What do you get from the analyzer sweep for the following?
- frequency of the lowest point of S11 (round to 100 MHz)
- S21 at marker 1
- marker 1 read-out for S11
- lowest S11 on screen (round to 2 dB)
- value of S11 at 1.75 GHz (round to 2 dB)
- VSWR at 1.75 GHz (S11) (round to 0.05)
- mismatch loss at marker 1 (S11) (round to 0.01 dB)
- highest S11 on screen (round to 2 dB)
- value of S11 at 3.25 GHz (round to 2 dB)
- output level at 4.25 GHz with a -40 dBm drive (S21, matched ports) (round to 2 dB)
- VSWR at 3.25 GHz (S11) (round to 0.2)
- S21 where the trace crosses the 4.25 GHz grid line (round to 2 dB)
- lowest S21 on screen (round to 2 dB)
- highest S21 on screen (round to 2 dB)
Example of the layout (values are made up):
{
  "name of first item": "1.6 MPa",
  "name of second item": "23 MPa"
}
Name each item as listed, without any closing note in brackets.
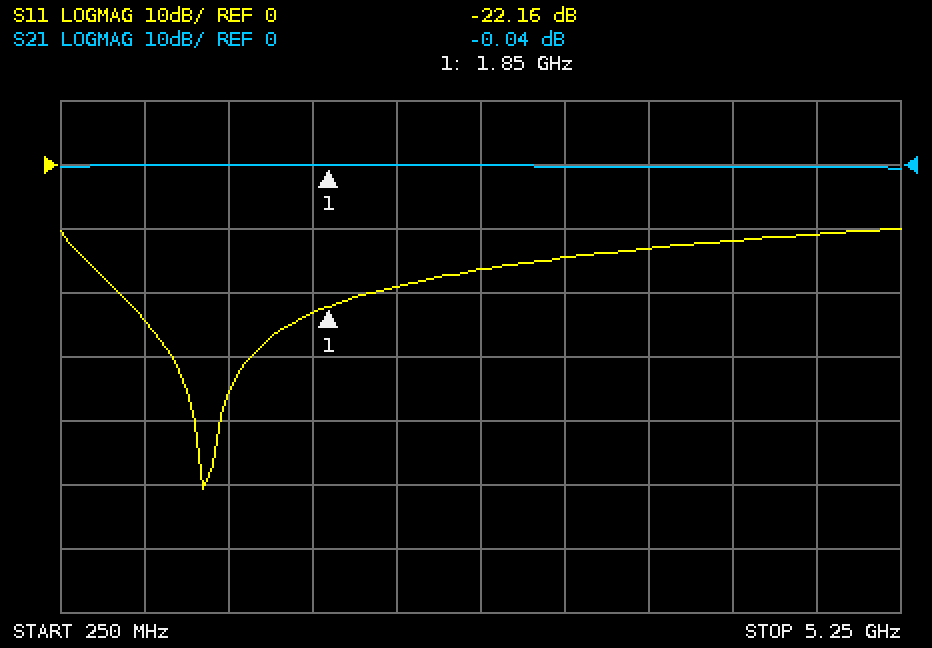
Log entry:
{
  "frequency of the lowest point of S11": "1.1 GHz",
  "S21 at marker 1": "-0.04 dB",
  "marker 1 read-out for S11": "-22.16 dB",
  "lowest S11 on screen": "-50 dB",
  "value of S11 at 1.75 GHz": "-24 dB",
  "VSWR at 1.75 GHz (S11)": "1.15",
  "mismatch loss at marker 1 (S11)": "0.03 dB",
  "highest S11 on screen": "-10 dB",
  "value of S11 at 3.25 GHz": "-14 dB",
  "output level at 4.25 GHz with a -40 dBm drive (S21, matched ports)": "-40 dBm",
  "VSWR at 3.25 GHz (S11)": "1.4",
  "S21 where the trace crosses the 4.25 GHz grid line": "0 dB",
  "lowest S21 on screen": "0 dB",
  "highest S21 on screen": "0 dB"
}
